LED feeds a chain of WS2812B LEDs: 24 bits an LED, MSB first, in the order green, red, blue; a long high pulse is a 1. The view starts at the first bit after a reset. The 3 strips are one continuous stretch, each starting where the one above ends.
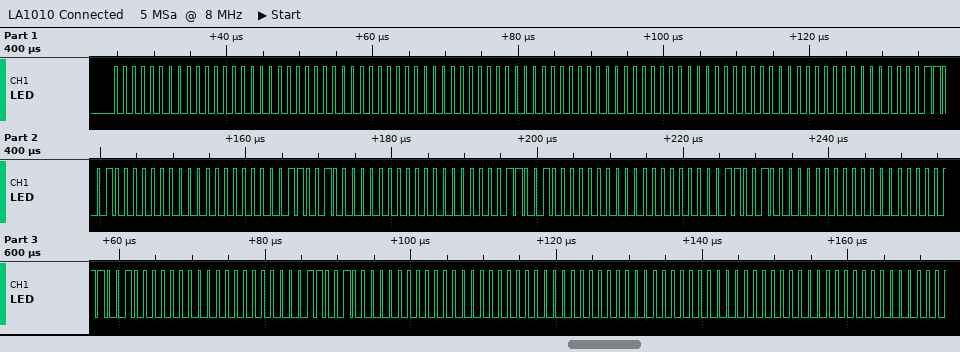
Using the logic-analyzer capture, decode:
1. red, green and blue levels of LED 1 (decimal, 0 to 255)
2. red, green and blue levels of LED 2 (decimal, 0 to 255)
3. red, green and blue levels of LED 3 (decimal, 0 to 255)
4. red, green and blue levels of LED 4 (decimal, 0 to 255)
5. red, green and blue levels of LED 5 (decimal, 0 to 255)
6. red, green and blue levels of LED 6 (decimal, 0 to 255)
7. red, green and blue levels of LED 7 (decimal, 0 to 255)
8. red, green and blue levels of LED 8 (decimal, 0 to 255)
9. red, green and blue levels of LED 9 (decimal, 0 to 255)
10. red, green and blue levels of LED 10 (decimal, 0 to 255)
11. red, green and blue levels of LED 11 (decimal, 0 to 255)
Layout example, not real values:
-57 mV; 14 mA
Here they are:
0, 0, 0; 0, 0, 0; 0, 0, 0; 0, 0, 100; 0, 0, 100; 0, 0, 100; 0, 0, 100; 0, 0, 100; 0, 0, 100; 0, 0, 0; 0, 0, 0
